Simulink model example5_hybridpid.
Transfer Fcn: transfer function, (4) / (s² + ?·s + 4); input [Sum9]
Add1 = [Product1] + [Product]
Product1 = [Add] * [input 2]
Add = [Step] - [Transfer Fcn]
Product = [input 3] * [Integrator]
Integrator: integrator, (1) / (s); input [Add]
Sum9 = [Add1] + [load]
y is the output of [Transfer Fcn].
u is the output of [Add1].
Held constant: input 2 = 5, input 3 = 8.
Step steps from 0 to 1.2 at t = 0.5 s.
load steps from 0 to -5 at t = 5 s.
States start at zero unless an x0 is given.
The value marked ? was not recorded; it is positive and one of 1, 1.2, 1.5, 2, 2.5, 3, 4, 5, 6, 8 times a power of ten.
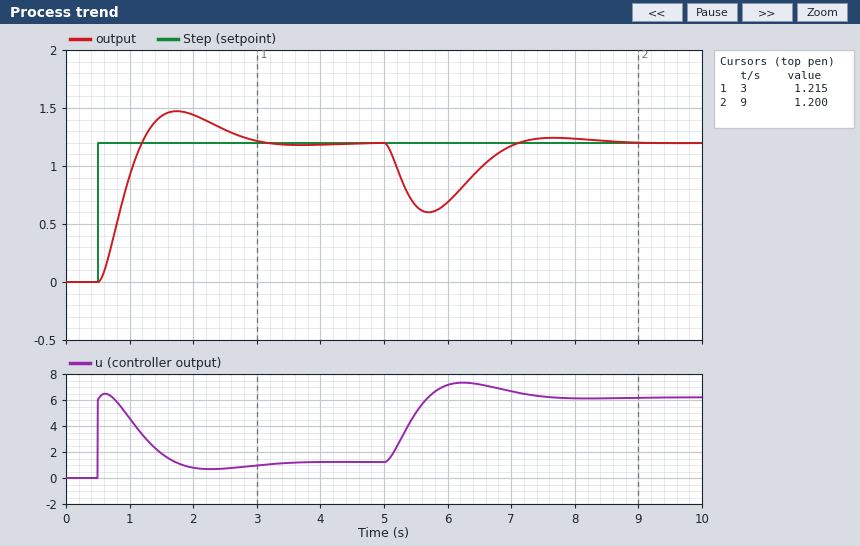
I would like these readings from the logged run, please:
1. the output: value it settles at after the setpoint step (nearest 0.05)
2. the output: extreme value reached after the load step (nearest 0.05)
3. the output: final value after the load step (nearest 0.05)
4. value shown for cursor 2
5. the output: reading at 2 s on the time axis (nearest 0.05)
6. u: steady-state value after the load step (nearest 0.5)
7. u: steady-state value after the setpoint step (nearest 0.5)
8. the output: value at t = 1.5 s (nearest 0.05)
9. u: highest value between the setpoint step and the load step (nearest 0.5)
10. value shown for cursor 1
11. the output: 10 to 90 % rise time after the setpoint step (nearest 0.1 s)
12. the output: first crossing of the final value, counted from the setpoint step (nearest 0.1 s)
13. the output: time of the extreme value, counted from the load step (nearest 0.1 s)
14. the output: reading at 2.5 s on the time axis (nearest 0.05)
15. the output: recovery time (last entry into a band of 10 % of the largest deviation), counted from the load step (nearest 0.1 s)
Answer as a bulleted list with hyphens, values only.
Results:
- 1.20
- 0.60
- 1.20
- 1.200
- 1.45
- 6.0
- 1.0
- 1.45
- 6.5
- 1.215
- 0.5 s
- 0.7 s
- 0.7 s
- 1.30
- 1.9 s
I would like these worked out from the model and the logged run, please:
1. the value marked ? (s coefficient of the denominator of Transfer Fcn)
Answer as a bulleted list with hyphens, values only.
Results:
- 10
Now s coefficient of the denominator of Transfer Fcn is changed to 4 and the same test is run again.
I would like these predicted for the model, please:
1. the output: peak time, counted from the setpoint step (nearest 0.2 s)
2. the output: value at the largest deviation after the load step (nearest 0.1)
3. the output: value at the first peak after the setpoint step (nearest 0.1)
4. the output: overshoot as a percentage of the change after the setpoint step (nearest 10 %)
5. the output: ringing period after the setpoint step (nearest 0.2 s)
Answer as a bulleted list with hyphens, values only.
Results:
- 0.8 s
- 0.3
- 1.7
- 40 %
- 1.4 s
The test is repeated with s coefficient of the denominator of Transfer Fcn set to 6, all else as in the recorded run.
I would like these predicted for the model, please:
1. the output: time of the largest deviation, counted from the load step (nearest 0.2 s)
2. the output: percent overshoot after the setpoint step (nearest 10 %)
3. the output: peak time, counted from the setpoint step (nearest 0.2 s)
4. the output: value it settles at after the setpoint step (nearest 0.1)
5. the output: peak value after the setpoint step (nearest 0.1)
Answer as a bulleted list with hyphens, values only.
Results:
- 0.6 s
- 30 %
- 0.8 s
- 1.2
- 1.5
